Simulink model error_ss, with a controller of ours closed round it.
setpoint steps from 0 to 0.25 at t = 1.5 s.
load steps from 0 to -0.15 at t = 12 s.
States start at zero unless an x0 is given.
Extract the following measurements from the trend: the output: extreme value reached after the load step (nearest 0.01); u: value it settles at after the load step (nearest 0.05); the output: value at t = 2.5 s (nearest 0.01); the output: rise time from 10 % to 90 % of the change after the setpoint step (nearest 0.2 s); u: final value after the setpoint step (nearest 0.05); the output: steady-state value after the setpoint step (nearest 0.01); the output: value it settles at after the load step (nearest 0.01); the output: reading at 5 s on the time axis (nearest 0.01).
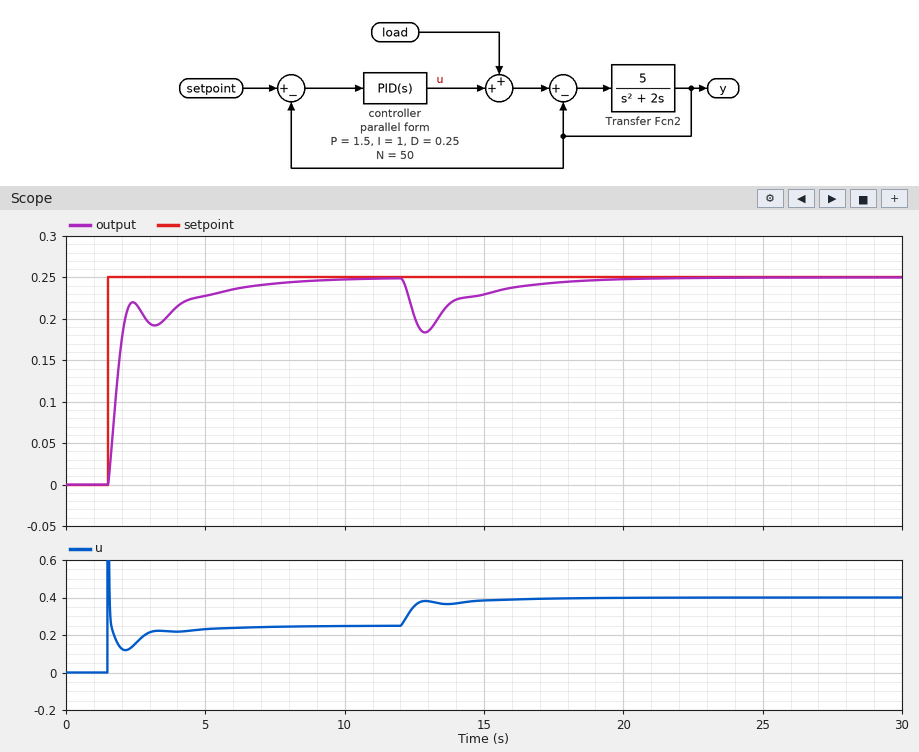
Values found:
0.18
0.40
0.22
3.0 s
0.25
0.25
0.25
0.23
